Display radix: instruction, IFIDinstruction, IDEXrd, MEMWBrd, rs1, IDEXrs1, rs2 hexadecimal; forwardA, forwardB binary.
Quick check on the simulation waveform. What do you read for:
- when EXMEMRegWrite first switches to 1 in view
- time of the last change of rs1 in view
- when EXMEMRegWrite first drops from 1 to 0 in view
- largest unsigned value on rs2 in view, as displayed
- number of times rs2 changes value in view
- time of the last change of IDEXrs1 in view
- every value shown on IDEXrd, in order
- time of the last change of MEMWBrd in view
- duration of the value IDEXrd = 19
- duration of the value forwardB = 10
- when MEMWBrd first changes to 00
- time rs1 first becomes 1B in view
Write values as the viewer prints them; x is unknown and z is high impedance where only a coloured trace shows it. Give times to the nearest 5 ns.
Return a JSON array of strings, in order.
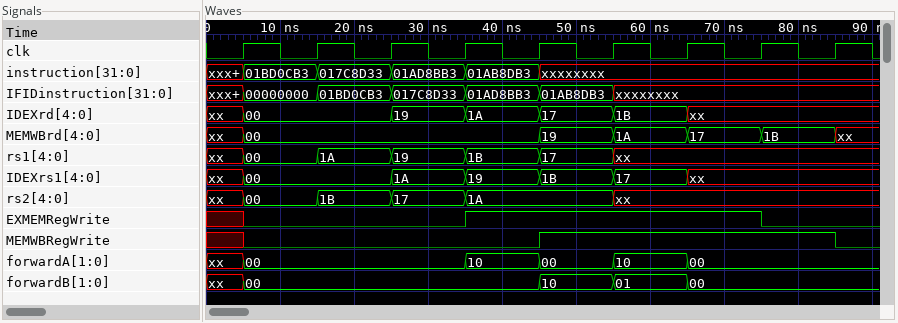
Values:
["35 ns", "55 ns", "75 ns", "1B", "5", "65 ns", "xx, 00, 19, 1A, 17, 1B, xx", "85 ns", "10 ns", "10 ns", "5 ns", "35 ns"]
